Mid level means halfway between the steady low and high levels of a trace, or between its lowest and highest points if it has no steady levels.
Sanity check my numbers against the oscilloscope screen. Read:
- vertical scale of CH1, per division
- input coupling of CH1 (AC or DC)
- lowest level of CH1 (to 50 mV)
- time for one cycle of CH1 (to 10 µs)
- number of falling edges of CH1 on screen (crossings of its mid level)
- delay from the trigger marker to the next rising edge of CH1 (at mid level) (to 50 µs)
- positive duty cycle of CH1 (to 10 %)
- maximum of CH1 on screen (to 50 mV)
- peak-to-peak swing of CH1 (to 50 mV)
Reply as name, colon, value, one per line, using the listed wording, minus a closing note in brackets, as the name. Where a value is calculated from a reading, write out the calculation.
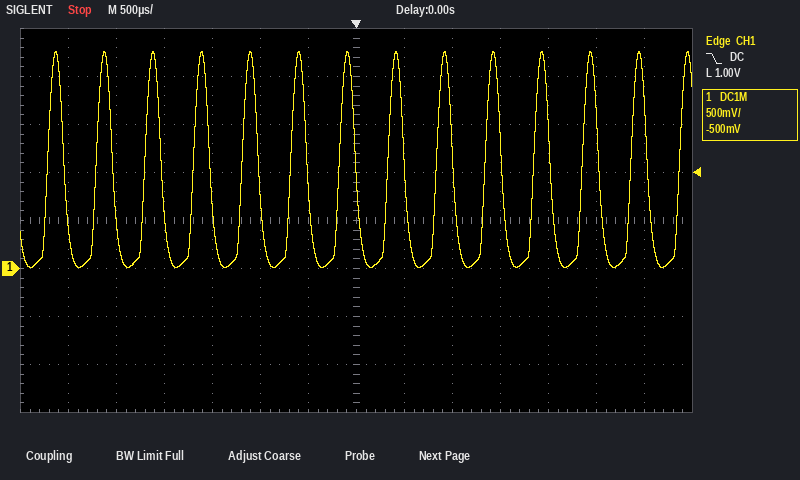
vertical scale of CH1, per division: 500 mV
input coupling of CH1: DC
lowest level of CH1: 0 mV
time for one cycle of CH1: 510 µs
number of falling edges of CH1 on screen: 13
delay from the trigger marker to the next rising edge of CH1 (at mid level): 350 µs
positive duty cycle of CH1: 30 %
maximum of CH1 on screen: 2.25 V
peak-to-peak swing of CH1: 2.25 V − (0 mV) = 2.25 V
